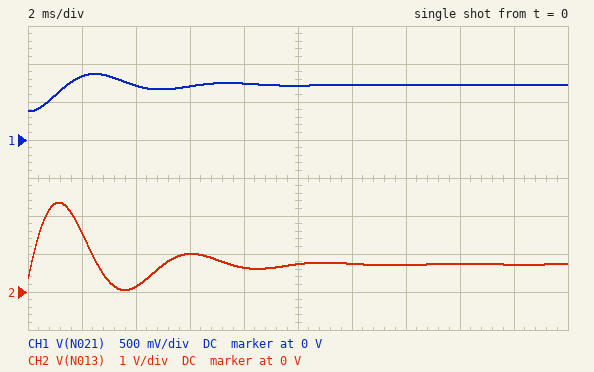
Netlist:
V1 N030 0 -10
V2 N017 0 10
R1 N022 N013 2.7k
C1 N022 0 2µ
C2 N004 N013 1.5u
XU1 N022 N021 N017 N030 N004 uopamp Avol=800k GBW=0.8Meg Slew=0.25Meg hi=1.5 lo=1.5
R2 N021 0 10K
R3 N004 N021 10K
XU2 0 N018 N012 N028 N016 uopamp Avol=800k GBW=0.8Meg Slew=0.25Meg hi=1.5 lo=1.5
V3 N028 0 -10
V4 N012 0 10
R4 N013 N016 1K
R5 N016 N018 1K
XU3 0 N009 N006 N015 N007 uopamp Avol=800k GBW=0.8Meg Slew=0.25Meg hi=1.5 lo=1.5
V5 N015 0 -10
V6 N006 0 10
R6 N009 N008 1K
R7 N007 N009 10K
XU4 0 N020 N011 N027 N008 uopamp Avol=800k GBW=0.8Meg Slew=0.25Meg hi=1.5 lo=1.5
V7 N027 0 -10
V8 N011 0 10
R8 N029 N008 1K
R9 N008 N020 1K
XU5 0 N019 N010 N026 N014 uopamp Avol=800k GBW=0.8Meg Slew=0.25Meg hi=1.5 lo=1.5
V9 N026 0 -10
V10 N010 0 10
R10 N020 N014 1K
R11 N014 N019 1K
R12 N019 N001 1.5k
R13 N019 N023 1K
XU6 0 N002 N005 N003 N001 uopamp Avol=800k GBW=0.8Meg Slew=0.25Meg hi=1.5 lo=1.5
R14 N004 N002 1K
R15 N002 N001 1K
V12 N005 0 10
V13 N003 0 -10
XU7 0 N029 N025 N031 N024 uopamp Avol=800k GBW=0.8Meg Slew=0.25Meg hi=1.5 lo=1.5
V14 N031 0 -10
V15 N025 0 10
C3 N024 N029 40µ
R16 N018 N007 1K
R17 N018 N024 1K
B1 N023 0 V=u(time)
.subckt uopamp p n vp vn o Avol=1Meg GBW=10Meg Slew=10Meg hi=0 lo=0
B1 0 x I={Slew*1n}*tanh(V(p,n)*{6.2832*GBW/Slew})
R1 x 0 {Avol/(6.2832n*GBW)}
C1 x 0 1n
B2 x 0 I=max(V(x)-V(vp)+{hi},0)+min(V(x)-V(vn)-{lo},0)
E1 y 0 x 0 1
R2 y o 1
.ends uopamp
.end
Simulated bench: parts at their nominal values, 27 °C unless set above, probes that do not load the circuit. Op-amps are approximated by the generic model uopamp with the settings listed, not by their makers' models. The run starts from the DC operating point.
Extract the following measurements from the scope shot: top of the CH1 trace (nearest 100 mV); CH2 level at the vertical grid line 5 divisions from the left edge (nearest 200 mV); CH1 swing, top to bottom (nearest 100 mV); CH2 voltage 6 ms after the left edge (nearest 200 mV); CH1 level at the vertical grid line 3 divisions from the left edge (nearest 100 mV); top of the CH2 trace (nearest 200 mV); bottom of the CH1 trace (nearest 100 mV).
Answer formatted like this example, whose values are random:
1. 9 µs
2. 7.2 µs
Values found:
1. 900 mV
2. 800 mV
3. 500 mV
4. 1.0 V
5. 700 mV
6. 2.4 V
7. 400 mV
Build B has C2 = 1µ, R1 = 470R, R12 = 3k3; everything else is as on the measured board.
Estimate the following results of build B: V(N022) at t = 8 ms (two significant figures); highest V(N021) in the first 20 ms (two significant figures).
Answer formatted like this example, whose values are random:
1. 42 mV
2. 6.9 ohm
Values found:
1. 1.5 V
2. 1.7 V
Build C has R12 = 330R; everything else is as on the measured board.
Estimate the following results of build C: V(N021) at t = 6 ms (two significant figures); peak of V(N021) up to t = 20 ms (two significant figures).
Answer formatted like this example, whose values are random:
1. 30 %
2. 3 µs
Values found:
1. 170 mV
2. 220 mV
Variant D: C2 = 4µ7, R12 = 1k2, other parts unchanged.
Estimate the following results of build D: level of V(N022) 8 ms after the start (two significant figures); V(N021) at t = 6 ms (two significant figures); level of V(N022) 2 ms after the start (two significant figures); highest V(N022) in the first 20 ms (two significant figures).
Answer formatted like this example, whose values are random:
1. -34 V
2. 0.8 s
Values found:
1. 400 mV
2. 540 mV
3. 590 mV
4. 820 mV
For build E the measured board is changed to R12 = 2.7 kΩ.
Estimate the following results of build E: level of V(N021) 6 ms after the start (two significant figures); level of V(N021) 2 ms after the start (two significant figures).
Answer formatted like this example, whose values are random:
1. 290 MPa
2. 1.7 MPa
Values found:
1. 1.2 V
2. 1.3 V
